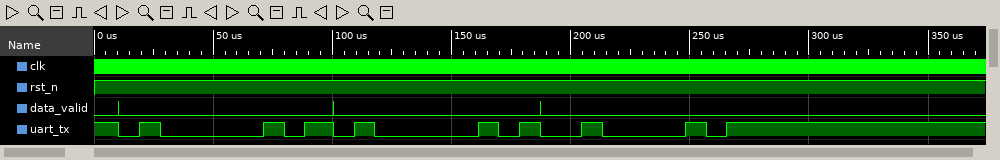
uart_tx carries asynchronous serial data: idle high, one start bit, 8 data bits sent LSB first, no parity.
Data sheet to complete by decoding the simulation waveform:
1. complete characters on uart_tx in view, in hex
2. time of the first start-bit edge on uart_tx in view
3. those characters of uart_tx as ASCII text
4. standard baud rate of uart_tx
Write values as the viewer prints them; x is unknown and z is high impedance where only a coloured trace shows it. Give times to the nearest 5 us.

41, 41, 42
10 us
"AAB"
115200 baud
